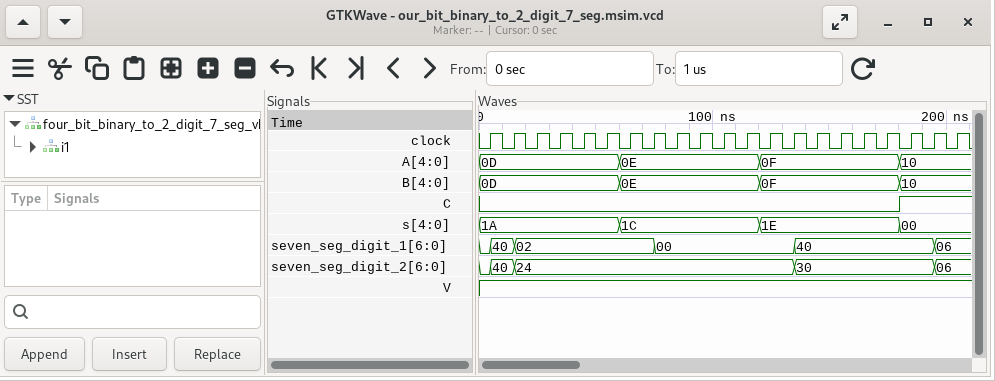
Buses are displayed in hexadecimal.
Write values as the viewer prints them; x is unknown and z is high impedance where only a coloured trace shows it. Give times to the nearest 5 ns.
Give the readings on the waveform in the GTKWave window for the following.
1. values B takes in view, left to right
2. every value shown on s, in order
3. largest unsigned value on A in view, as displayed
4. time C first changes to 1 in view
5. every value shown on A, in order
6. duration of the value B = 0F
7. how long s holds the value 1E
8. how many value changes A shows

0D, 0E, 0F, 10
1A, 1C, 1E, 00
10
180 ns
0D, 0E, 0F, 10
60 ns
60 ns
3
